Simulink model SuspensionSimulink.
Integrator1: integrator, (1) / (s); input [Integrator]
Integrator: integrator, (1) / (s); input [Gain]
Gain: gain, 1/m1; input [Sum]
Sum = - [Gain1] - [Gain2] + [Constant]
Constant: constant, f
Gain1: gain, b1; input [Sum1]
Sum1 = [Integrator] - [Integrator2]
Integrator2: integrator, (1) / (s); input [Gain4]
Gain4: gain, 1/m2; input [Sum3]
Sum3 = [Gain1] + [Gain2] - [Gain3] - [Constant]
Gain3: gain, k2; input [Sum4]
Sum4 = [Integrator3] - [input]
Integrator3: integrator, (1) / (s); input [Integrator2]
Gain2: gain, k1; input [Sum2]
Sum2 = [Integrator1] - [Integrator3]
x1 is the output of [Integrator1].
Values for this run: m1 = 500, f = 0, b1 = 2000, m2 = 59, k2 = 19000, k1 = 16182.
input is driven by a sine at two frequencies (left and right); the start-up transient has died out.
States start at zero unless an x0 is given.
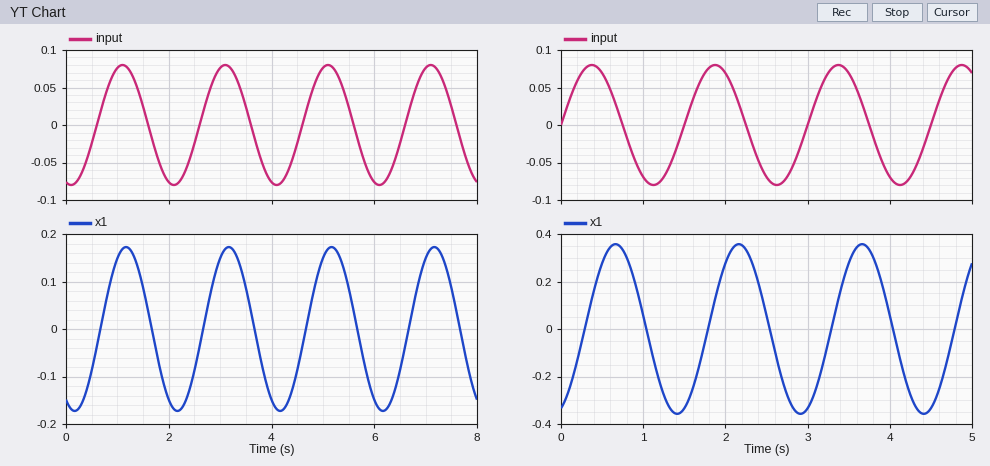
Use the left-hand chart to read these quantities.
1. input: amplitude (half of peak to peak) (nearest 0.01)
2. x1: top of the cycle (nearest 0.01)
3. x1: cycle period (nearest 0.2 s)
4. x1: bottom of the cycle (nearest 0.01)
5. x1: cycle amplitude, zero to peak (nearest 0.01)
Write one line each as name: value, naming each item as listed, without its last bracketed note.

input: amplitude (half of peak to peak): 0.08
x1: top of the cycle: 0.17
x1: cycle period: 2.0 s
x1: bottom of the cycle: -0.17
x1: cycle amplitude, zero to peak: 0.17
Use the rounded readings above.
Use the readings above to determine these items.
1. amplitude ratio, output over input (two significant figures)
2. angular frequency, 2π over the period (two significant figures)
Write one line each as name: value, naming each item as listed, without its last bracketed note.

amplitude ratio, output over input: 2.1
angular frequency, 2π over the period: 3.1 rad/s
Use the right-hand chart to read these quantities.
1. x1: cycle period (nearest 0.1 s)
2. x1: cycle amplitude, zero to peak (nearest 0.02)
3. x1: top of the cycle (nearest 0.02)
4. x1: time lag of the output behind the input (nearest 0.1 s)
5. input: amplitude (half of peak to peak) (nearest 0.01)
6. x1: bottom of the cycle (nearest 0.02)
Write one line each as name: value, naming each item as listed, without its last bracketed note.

x1: cycle period: 1.5 s
x1: cycle amplitude, zero to peak: 0.36
x1: top of the cycle: 0.36
x1: time lag of the output behind the input: 0.3 s
input: amplitude (half of peak to peak): 0.08
x1: bottom of the cycle: -0.36
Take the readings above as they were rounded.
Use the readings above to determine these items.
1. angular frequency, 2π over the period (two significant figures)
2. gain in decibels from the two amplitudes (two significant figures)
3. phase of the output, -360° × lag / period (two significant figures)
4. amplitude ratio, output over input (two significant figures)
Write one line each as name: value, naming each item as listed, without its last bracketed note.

angular frequency, 2π over the period: 4.2 rad/s
gain in decibels from the two amplitudes: 13 dB
phase of the output, -360° × lag / period: -72°
amplitude ratio, output over input: 4.5
